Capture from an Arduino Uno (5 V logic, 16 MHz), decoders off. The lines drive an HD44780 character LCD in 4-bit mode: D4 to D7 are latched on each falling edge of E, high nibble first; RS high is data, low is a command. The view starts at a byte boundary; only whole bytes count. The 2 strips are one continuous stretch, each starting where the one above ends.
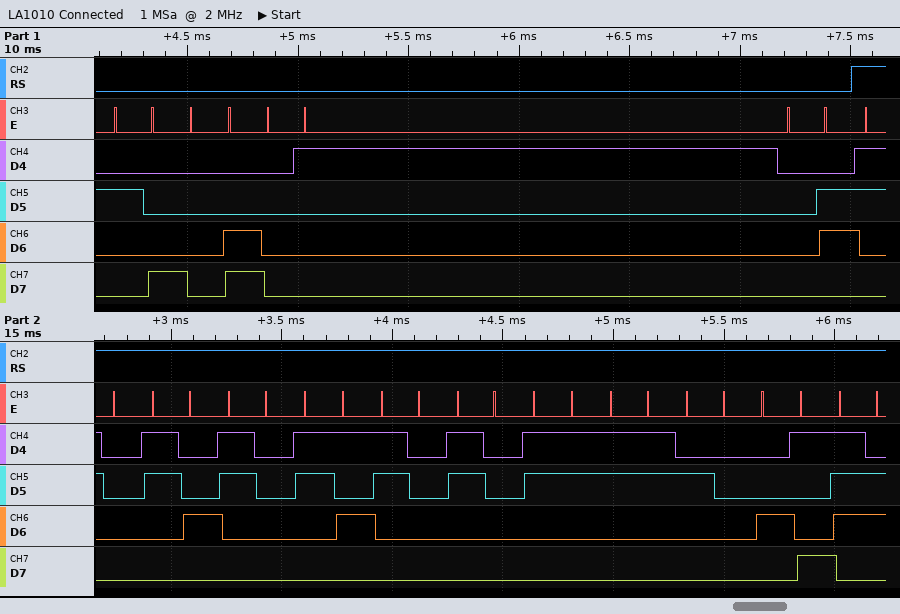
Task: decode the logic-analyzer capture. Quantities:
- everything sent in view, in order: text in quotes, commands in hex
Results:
0x28 0x0C 0x01 0x06 "04050033 Iv"
